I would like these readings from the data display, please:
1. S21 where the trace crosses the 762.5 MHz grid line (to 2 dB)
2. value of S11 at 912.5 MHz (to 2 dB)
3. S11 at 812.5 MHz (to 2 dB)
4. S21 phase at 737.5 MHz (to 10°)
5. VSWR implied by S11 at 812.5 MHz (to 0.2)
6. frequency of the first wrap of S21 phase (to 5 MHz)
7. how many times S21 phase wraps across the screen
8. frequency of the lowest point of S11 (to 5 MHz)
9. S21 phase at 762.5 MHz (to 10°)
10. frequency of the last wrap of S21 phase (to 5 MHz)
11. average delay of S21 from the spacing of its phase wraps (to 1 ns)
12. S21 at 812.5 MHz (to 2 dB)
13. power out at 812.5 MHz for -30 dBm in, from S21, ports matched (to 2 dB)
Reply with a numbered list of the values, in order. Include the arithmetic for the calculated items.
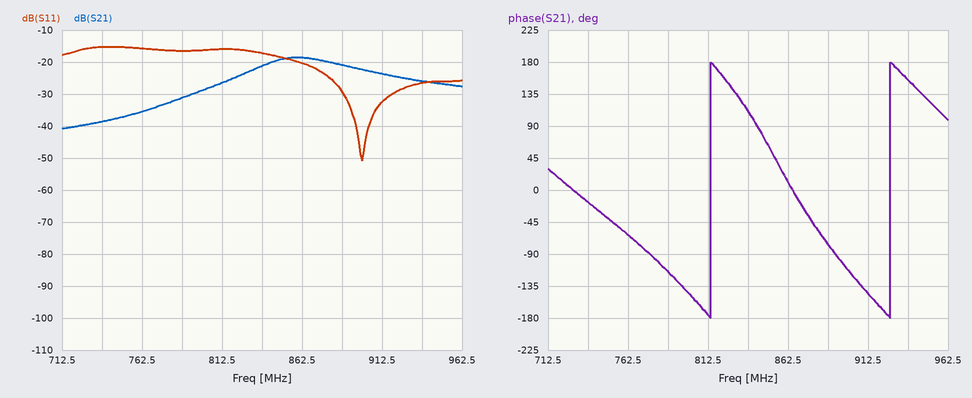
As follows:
1. -36 dB
2. -32 dB
3. -16 dB
4. -20°
5. |Γ| = 10^(-16/20) = 0.1585; VSWR = (1 + 0.1585)/(1 − 0.1585) ≈ 1.4
6. 815 MHz
7. 2
8. 900 MHz
9. -60°
10. 925 MHz
11. 1 cycle / (925 MHz − 815 MHz) ≈ 9 ns
12. -26 dB
13. -30 dBm + (-26 dB) = -56 dBm
